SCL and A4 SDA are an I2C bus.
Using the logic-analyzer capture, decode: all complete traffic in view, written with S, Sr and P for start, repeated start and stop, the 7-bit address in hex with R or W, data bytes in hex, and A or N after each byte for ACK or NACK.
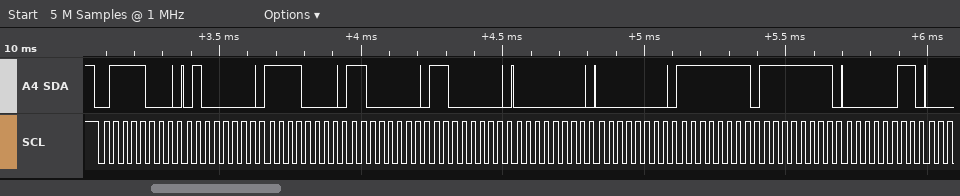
S 3CW A 40 A F0 A C0 A C0 A 00 A 00 A FF A FF A 03 A
